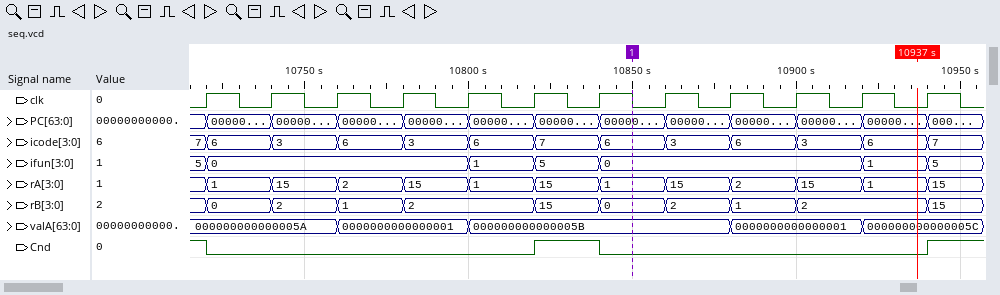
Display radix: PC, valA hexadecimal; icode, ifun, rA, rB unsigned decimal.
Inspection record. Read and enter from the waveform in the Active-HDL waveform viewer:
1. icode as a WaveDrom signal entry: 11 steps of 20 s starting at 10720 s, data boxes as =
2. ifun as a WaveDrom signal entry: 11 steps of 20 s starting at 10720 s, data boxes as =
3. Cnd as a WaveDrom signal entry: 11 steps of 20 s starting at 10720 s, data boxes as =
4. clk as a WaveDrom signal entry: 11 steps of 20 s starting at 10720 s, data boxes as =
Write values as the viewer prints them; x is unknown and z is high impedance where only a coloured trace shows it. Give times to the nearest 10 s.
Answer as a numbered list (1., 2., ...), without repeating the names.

1. {name: 'icode', wave: '===========', data: '6 3 6 3 6 7 6 3 6 3 6'}
2. {name: 'ifun', wave: '=...===...=', data: '0 1 5 0 1'}
3. {name: 'Cnd', wave: '0....10....'}
4. {name: 'clk', wave: 'p..........'}
